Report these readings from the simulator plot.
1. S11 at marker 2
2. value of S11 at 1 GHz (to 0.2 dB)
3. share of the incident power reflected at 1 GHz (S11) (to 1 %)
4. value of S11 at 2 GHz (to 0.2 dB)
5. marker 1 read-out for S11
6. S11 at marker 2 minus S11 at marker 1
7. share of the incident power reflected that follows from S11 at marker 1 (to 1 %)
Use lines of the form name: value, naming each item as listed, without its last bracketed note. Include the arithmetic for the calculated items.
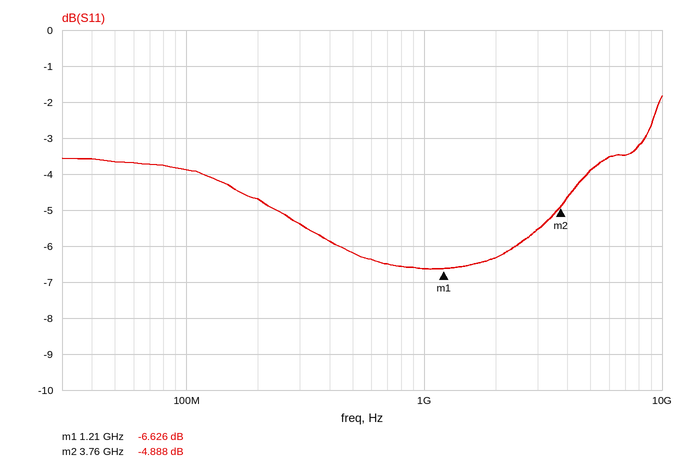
S11 at marker 2: -4.888 dB
value of S11 at 1 GHz: -6.6 dB
share of the incident power reflected at 1 GHz (S11): 10^(-6.6/10) ≈ 22 %
value of S11 at 2 GHz: -6.4 dB
marker 1 read-out for S11: -6.626 dB
S11 at marker 2 minus S11 at marker 1: -4.888 − (-6.626) = 1.738 dB
share of the incident power reflected that follows from S11 at marker 1: 10^(-6.626/10) ≈ 22 %
